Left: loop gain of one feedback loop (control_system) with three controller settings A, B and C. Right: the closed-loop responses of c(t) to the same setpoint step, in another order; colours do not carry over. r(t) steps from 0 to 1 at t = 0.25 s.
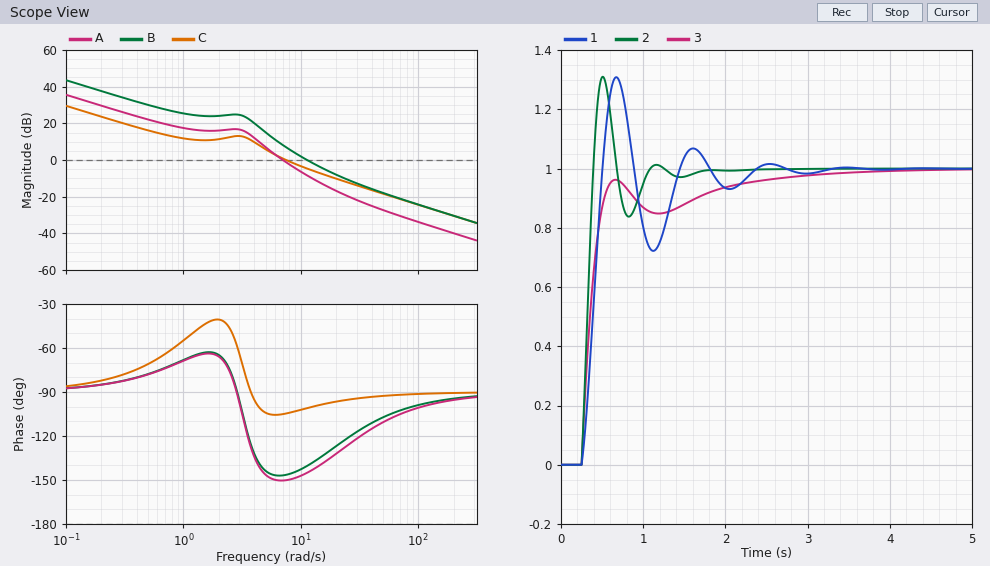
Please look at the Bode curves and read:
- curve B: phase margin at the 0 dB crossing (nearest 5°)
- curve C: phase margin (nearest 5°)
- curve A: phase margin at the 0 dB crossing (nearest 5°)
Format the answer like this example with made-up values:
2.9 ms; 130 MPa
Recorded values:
40°; 75°; 30°
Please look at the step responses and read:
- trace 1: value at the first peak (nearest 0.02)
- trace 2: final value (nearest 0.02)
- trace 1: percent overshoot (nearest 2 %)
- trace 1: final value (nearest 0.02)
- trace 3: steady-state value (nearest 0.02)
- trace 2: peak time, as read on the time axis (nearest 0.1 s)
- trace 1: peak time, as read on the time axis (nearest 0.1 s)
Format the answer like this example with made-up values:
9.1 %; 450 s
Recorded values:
1.30; 1.00; 30 %; 1.00; 1.00; 0.5 s; 0.7 s
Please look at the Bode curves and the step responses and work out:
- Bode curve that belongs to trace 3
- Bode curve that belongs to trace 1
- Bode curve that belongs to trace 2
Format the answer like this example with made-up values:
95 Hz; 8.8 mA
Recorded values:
C; A; B
